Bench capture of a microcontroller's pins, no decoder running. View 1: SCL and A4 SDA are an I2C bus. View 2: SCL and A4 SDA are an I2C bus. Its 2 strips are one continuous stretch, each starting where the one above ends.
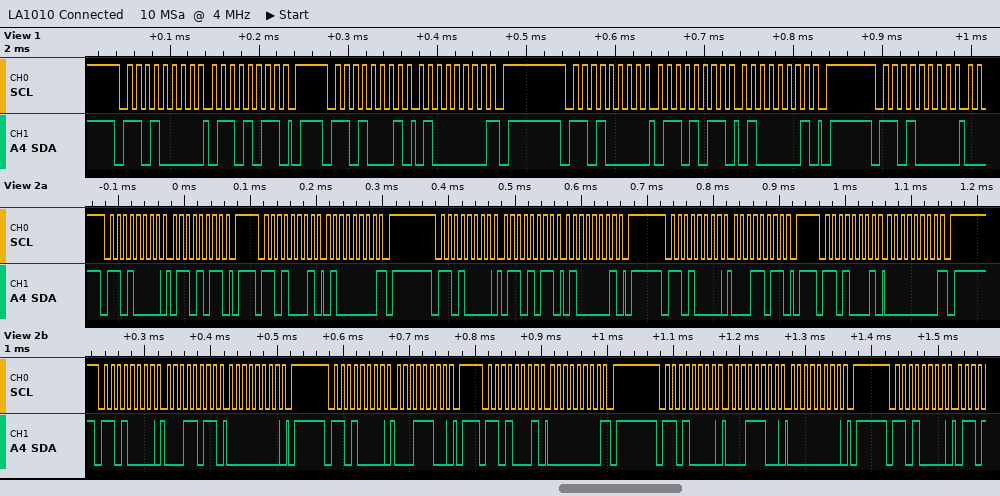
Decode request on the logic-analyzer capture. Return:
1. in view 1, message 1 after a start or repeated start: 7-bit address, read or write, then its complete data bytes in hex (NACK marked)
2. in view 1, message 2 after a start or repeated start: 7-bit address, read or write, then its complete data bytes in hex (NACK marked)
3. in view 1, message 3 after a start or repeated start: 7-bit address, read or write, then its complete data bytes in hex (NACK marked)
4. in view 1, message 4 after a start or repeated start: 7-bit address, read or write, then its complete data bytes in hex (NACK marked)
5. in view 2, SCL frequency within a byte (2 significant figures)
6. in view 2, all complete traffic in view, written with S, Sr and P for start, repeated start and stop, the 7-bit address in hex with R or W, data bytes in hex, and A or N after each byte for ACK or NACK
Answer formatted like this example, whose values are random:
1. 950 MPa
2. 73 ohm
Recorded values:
1. 0x68 write: 6B
2. 0x68 read: 40 NACK
3. 0x68 write: 6B 41
4. 0x68 write
5. 100 kHz
6. S 68W A 6B A P S 68R A 40 N P S 68W A 6B A 41 A P S 68W A 1B A P S 68R A 00 N P S 68W A 1B A 00 A P S 68W A 1C A P S 68R A 00 N P S 68W A 1C A 00 A P S 68W A
